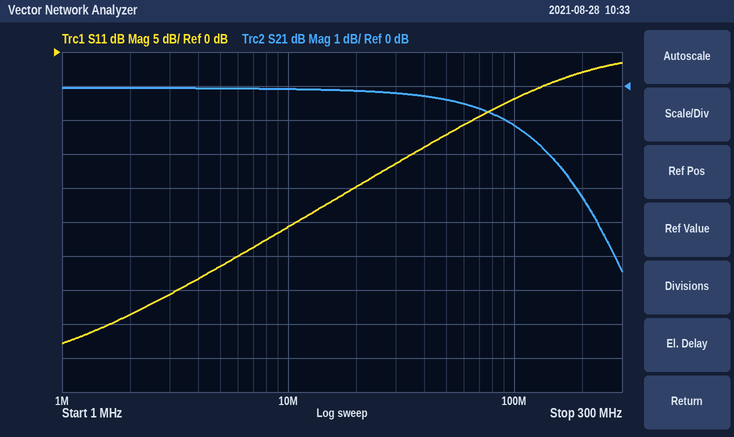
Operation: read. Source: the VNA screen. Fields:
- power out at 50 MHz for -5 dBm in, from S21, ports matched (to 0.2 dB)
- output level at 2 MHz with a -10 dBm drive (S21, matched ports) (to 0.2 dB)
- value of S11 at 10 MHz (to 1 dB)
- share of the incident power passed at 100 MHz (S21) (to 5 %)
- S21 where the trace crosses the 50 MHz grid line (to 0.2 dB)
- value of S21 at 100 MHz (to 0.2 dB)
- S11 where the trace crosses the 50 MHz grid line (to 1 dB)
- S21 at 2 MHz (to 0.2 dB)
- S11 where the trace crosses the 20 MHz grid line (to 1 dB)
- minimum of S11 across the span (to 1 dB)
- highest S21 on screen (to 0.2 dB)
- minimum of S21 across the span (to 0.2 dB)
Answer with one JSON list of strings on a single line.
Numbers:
["-5.4 dBm", "-10.0 dBm", "-26 dB", "75 %", "-0.4 dB", "-1.2 dB", "-12 dB", "0.0 dB", "-20 dB", "-43 dB", "0.0 dB", "-5.4 dB"]
